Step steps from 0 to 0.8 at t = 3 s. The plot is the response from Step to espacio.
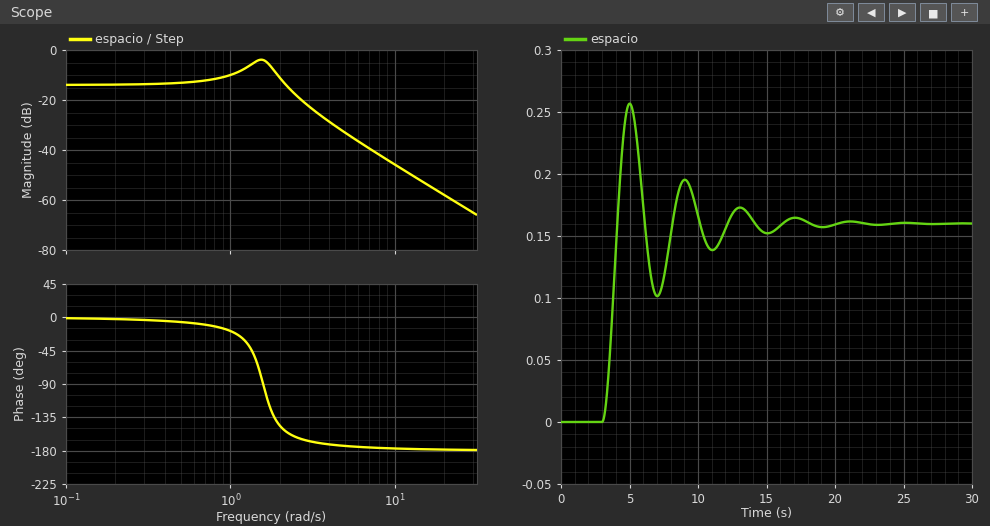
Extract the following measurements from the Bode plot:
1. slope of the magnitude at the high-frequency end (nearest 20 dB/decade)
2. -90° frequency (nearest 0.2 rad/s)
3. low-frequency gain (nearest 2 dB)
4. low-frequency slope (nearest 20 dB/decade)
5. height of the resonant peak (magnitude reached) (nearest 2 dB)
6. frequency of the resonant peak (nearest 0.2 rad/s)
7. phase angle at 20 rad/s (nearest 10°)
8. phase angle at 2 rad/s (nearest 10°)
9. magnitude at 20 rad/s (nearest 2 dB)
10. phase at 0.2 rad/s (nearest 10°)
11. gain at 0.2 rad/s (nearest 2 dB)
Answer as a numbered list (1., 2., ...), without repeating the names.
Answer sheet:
1. -40 dB/decade
2. 1.6 rad/s
3. -14 dB
4. 0 dB/decade
5. -4 dB
6. 1.6 rad/s
7. -180°
8. -150°
9. -58 dB
10. 0°
11. -14 dB
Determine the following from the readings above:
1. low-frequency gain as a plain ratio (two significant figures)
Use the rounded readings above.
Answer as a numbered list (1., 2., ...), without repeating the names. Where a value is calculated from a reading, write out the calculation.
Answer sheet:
1. 10^(-14 / 20) = 0.20
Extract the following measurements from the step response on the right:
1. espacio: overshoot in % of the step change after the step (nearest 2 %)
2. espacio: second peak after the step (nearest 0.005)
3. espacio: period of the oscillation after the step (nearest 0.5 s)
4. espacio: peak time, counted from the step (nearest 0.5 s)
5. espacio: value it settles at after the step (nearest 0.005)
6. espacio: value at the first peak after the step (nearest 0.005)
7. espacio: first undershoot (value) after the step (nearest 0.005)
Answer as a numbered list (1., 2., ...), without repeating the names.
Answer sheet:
1. 60 %
2. 0.195
3. 4.0 s
4. 2.0 s
5. 0.160
6. 0.255
7. 0.100
